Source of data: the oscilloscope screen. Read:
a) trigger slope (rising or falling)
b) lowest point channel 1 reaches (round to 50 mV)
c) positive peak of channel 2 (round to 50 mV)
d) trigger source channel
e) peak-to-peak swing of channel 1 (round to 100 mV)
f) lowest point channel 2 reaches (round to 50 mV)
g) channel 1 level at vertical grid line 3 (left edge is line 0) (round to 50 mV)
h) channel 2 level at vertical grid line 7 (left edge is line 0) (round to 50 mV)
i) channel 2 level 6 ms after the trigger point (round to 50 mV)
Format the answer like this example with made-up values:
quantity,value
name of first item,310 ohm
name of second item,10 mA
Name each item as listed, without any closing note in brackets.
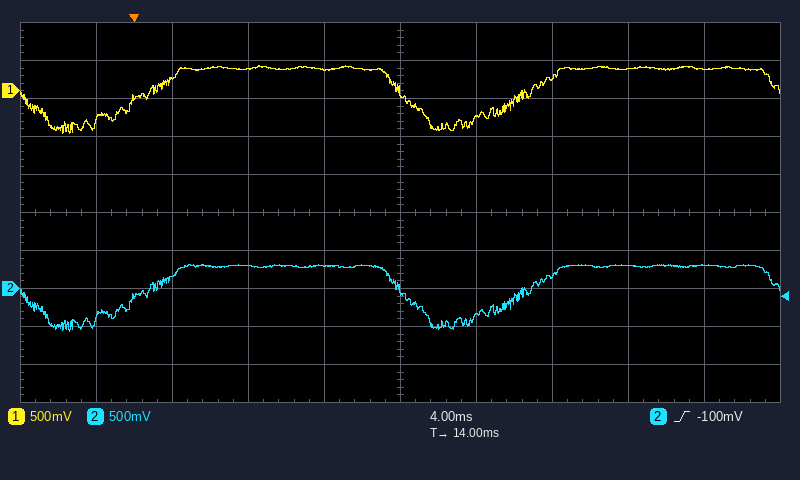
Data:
quantity,value
trigger slope,rising
lowest point channel 1 reaches,-550 mV
positive peak of channel 2,300 mV
trigger source channel,channel 2
peak-to-peak swing of channel 1,900 mV
lowest point channel 2 reaches,-550 mV
channel 1 level at vertical grid line 3 (left edge is line 0),300 mV
channel 2 level at vertical grid line 7 (left edge is line 0),150 mV
channel 2 level 6 ms after the trigger point,300 mV
